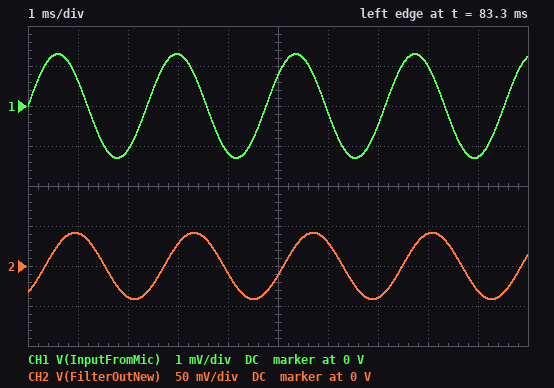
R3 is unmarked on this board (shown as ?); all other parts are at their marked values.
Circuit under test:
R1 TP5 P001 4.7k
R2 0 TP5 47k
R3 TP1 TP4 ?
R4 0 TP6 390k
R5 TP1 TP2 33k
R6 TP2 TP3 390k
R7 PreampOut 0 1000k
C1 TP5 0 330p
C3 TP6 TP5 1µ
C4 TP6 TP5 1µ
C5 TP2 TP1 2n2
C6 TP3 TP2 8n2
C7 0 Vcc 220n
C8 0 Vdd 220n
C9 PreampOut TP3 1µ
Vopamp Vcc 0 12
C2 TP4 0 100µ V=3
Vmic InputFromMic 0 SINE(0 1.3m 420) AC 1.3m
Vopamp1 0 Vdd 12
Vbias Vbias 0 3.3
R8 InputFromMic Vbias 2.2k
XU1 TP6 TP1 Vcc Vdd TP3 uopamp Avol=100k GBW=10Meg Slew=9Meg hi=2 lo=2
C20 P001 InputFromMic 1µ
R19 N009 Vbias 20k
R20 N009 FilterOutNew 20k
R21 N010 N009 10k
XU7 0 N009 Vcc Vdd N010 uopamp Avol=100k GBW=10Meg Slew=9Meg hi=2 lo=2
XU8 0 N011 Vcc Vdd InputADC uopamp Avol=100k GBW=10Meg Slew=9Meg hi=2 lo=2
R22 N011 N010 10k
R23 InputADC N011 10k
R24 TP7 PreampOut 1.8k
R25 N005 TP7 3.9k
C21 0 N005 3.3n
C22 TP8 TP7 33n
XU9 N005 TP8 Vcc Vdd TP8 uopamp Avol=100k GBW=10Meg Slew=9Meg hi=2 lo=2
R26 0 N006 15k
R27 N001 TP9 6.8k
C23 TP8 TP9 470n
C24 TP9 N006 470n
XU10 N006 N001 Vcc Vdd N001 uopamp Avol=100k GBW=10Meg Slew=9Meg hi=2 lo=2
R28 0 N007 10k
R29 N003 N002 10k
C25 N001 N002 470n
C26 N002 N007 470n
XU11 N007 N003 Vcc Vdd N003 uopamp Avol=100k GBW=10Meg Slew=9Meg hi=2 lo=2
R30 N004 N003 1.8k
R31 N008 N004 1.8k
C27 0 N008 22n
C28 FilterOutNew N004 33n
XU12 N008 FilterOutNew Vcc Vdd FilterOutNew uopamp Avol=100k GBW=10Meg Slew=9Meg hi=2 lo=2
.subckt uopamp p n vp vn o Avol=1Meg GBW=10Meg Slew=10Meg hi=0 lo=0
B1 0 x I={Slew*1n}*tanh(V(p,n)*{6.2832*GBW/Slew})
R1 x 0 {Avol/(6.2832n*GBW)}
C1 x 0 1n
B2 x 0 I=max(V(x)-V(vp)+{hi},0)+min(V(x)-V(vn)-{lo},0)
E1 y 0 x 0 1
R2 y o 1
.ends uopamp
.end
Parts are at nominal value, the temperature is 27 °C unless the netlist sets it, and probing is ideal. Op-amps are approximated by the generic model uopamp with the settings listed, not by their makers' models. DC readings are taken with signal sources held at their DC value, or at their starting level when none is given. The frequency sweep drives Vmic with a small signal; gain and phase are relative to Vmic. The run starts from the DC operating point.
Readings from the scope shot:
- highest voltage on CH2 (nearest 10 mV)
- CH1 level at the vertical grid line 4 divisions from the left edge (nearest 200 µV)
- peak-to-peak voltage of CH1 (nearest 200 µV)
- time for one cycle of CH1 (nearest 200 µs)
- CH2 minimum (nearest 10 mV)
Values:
40 mV
-1.2 mV
2.6 mV
2.4 ms
-40 mV
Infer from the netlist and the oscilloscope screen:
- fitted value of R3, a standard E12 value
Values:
1.8 kΩ
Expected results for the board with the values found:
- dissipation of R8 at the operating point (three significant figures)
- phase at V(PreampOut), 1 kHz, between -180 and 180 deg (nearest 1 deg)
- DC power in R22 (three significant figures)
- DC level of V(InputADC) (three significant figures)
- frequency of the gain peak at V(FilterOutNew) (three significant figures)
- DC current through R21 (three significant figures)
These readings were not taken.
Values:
4.95 mW
-47 deg
272 µW
1.65 V
61.4 Hz
165 µA
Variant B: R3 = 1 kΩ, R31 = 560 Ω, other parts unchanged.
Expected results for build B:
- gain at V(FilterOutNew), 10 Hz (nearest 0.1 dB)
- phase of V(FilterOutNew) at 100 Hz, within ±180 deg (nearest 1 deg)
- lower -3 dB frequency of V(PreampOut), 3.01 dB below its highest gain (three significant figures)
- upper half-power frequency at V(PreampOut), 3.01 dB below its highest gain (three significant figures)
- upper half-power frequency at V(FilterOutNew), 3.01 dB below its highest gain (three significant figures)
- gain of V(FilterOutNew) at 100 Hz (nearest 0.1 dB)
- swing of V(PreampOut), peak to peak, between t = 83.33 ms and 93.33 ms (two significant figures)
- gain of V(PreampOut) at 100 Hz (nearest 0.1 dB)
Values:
7.9 dB
10 deg
3.58 Hz
57.6 Hz
135 Hz
43.8 dB
150 mV
44.7 dB
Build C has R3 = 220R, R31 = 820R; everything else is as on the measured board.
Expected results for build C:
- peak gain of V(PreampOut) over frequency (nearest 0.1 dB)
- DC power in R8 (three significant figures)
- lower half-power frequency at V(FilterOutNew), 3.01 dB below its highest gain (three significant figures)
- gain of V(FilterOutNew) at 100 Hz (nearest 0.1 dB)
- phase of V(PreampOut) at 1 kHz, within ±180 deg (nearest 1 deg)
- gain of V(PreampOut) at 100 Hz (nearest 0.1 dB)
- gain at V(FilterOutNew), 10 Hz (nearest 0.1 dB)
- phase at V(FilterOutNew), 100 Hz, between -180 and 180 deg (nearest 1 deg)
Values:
63.3 dB
4.95 mW
36.2 Hz
56.8 dB
-49 deg
57.7 dB
19.2 dB
13 deg
